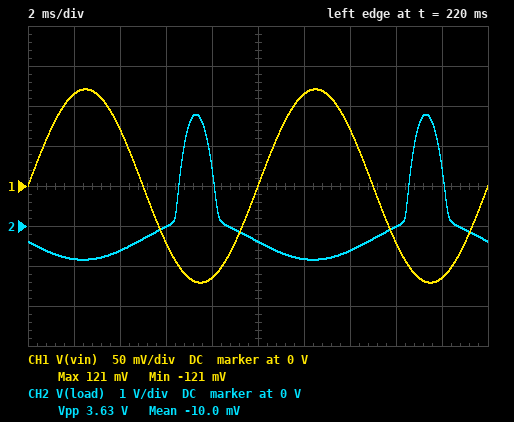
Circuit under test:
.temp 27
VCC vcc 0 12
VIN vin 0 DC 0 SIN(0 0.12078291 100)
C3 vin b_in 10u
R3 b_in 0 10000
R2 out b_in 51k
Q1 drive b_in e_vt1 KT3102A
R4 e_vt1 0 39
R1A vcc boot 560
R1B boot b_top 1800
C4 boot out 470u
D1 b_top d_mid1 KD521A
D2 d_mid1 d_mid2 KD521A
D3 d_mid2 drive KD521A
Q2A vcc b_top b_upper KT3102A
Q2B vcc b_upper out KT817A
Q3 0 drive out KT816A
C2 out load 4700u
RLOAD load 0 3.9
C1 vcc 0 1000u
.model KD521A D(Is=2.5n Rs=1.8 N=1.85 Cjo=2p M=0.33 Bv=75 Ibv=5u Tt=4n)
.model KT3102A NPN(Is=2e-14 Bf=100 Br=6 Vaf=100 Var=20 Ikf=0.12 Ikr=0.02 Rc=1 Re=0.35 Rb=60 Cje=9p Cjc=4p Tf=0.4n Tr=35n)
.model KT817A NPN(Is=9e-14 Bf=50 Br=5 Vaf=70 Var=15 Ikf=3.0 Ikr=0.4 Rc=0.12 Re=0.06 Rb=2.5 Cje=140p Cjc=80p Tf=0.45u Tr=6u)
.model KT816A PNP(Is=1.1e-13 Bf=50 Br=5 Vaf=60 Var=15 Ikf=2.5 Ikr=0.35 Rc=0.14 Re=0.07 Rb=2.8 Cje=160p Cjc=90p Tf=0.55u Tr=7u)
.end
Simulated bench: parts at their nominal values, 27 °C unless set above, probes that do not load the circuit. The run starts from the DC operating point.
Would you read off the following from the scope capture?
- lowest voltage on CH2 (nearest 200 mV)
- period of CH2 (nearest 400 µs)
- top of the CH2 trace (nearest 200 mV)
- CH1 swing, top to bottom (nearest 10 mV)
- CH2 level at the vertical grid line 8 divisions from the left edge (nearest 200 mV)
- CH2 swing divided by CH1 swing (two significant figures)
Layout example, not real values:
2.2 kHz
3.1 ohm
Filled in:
-800 mV
10.0 ms
2.8 V
240 mV
0 V
15
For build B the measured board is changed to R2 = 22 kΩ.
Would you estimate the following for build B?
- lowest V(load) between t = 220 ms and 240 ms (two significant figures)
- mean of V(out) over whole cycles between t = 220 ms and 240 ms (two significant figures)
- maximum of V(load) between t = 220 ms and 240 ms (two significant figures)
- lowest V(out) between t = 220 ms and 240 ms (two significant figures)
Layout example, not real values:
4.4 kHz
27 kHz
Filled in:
-820 mV
4.0 V
2.7 V
3.2 V
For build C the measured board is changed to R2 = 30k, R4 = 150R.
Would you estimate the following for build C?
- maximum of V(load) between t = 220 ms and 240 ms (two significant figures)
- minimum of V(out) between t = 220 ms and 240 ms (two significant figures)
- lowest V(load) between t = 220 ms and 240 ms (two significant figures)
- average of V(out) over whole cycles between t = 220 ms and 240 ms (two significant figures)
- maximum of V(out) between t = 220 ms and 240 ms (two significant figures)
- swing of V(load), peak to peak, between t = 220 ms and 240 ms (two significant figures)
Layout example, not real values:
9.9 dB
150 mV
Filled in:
480 mV
5.1 V
-220 mV
5.4 V
5.8 V
700 mV
